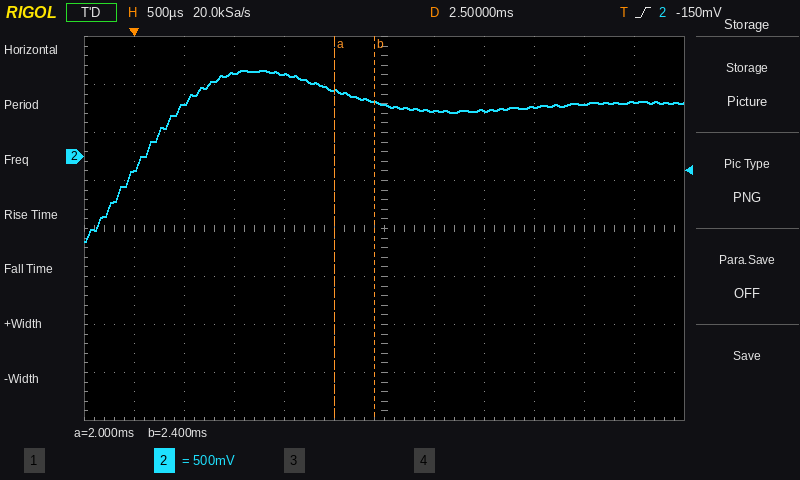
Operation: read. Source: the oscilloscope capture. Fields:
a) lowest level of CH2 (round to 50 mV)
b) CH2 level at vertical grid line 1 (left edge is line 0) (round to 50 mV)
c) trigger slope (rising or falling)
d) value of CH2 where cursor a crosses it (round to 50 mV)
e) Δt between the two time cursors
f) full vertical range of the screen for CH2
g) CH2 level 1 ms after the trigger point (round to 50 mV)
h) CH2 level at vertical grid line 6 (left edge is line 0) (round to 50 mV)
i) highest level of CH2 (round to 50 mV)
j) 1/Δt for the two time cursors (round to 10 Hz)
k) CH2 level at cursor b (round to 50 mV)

-900 mV
-150 mV
rising
700 mV
400 µs
4 V
850 mV
550 mV
900 mV
2.50 kHz
550 mV
